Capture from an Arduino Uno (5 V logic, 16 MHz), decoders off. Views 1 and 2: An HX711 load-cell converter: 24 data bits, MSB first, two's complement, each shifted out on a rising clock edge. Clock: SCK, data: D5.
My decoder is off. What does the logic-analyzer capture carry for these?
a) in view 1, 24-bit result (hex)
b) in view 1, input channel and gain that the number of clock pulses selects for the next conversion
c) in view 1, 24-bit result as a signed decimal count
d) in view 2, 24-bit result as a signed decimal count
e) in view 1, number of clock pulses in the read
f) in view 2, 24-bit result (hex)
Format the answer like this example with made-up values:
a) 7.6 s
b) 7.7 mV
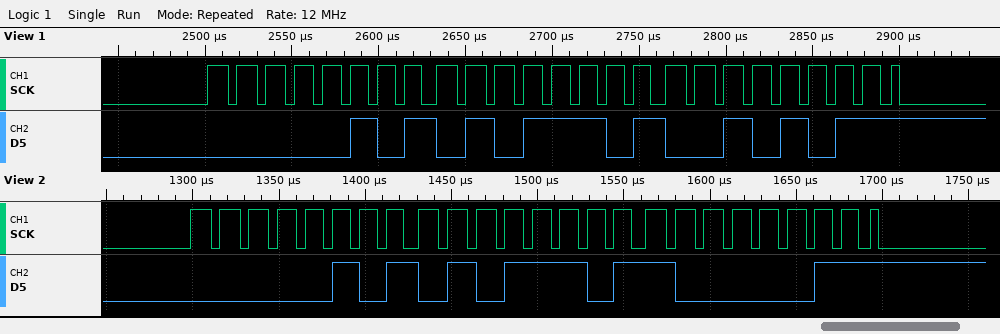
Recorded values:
a) 0x055D2B
b) channel A, gain 128
c) 351531
d) 351619
e) 25
f) 0x055D83
